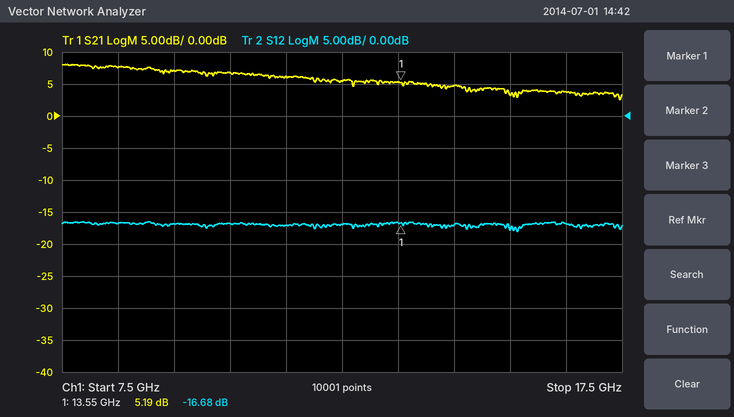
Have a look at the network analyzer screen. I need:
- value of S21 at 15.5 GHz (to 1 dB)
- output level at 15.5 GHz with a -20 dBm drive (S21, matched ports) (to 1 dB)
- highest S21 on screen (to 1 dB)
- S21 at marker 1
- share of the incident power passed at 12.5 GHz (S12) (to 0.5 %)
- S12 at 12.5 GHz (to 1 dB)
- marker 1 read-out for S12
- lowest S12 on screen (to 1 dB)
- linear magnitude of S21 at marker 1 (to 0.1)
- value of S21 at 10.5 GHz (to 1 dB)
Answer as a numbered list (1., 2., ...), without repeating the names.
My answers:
1. 3 dB
2. -17 dBm
3. 8 dB
4. 5.19 dB
5. 2.0 %
6. -17 dB
7. -16.68 dB
8. -18 dB
9. 1.8
10. 7 dB
